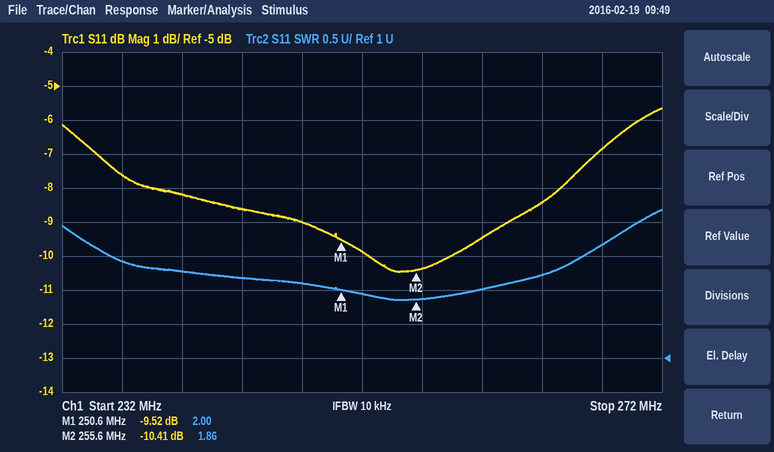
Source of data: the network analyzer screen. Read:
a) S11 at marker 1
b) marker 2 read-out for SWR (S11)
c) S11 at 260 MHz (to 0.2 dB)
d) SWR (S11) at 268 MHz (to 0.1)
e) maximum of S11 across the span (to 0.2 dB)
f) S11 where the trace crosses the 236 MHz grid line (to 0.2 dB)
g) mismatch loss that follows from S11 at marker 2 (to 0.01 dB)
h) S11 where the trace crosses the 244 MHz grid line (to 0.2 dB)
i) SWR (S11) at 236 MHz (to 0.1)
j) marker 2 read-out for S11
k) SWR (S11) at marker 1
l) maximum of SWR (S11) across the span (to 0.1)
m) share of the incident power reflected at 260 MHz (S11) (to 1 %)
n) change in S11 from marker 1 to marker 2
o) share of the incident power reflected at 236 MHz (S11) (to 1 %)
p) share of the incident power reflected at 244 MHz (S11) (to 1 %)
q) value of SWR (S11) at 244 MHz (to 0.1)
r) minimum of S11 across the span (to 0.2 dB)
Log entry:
-9.52 dB
1.86
-9.4 dB
2.7
-5.6 dB
-7.6 dB
0.41 dB
-8.6 dB
2.4
-10.41 dB
2.00
3.2
11 %
-0.89 dB
17 %
14 %
2.2
-10.4 dB
